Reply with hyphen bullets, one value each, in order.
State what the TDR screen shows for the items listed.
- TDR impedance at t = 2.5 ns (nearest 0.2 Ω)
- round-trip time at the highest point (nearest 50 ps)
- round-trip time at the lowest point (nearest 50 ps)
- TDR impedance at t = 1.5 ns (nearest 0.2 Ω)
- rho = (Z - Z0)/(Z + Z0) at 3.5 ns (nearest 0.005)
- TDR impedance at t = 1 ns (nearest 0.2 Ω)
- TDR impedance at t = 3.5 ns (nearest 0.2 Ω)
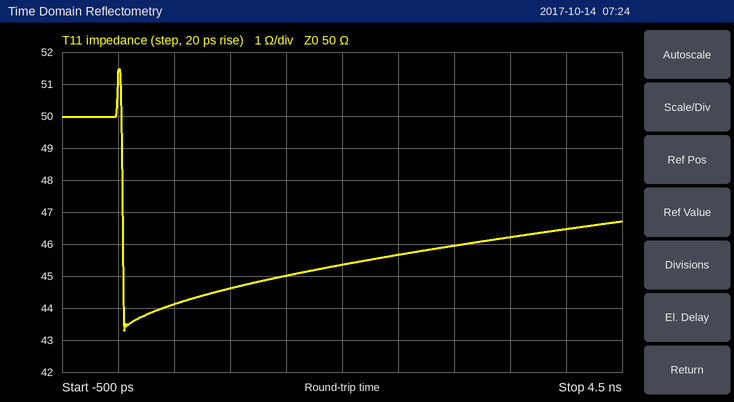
- 45.6 Ω
- 0 ps
- 50 ps
- 45.0 Ω
- -0.040
- 44.6 Ω
- 46.2 Ω
